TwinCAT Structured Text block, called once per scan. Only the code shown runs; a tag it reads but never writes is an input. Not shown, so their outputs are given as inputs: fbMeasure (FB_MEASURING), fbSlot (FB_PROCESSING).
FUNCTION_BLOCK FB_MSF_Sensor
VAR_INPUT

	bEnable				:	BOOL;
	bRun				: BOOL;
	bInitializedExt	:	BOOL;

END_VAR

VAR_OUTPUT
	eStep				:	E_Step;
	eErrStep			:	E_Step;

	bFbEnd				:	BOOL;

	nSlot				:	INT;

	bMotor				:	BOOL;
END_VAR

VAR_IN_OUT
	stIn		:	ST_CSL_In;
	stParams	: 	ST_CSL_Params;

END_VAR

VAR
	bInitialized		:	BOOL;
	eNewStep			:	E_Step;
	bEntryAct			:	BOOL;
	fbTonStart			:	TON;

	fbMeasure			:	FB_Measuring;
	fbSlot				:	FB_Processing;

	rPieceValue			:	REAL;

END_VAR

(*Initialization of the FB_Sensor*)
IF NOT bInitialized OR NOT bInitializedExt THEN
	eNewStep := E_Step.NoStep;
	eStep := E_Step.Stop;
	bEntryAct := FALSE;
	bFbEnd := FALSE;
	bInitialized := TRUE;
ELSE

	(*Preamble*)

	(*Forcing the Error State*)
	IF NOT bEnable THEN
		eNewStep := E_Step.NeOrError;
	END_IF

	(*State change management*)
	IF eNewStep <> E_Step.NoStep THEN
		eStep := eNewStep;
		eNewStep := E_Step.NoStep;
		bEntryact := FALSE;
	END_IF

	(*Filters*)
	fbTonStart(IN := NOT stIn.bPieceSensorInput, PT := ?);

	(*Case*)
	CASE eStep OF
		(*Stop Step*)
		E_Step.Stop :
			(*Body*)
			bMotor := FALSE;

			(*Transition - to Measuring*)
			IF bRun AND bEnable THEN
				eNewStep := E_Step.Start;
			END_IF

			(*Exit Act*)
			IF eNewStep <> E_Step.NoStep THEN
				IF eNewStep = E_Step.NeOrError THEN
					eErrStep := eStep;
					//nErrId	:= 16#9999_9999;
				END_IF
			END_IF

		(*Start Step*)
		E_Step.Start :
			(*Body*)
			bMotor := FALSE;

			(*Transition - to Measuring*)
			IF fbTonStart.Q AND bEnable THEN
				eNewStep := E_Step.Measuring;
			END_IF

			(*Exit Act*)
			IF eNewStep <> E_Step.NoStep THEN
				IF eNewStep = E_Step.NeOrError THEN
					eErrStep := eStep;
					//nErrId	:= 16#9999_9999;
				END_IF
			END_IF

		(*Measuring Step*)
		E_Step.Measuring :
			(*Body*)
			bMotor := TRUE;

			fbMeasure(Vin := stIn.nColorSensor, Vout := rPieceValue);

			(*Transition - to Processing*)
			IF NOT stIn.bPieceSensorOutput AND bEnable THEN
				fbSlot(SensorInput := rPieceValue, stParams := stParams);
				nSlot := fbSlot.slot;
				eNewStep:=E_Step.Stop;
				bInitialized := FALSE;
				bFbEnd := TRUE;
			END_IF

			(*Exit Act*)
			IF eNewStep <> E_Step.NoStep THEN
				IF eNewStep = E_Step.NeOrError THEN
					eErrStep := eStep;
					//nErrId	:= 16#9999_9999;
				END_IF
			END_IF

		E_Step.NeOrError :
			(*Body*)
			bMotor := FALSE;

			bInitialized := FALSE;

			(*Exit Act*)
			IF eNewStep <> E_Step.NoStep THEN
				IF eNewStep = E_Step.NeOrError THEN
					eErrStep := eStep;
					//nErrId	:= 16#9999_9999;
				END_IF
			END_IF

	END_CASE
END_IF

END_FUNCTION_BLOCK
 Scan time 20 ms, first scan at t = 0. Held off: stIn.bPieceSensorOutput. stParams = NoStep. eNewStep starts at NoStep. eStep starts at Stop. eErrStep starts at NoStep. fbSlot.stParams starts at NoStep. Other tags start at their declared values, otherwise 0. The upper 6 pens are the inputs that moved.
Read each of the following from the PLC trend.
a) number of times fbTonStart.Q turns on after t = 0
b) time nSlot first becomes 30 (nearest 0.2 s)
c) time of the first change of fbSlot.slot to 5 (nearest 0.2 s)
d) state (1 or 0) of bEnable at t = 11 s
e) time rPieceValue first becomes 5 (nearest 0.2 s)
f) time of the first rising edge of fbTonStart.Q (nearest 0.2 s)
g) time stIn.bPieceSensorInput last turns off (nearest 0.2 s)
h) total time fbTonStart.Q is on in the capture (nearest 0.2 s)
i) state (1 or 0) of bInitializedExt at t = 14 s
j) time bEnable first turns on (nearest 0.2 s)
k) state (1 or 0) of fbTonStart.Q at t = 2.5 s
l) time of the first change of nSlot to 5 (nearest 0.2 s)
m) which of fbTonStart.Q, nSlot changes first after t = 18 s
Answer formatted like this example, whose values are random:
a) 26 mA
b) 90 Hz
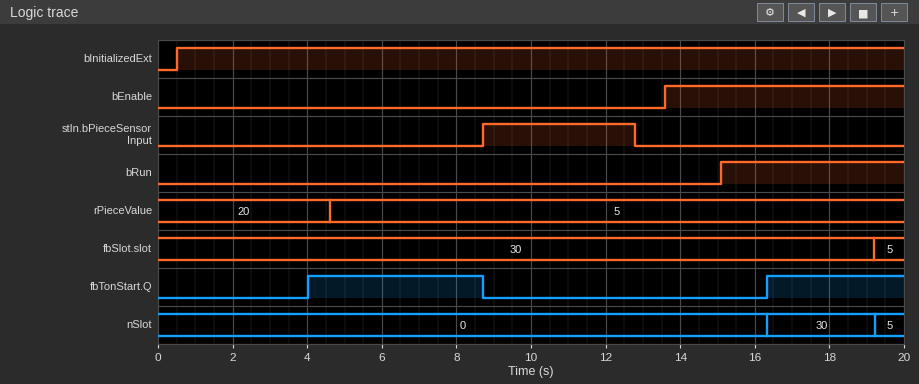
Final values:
a) 2
b) 16.4 s
c) 19.2 s
d) 0
e) 4.6 s
f) 4.0 s
g) 12.8 s
h) 8.4 s
i) 1
j) 13.6 s
k) 0
l) 19.2 s
m) nSlot
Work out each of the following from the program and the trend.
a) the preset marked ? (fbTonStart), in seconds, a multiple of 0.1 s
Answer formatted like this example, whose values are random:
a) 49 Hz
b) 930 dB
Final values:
a) 3.5 s
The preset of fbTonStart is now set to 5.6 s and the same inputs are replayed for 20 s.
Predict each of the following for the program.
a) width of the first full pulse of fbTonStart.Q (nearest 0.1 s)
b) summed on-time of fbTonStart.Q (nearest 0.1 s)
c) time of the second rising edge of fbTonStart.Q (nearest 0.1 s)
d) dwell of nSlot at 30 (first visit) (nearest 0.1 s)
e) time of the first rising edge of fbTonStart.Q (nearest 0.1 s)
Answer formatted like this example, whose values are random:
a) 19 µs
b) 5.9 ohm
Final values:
a) 2.6 s
b) 4.2 s
c) 18.4 s
d) 0.8 s
e) 6.1 s
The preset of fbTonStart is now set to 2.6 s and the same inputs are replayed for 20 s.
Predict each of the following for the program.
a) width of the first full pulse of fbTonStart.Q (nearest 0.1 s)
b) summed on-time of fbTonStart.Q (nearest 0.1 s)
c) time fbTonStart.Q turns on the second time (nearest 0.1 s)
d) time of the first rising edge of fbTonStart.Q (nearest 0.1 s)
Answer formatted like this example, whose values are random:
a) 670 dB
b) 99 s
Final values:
a) 5.6 s
b) 10.2 s
c) 15.4 s
d) 3.1 s
